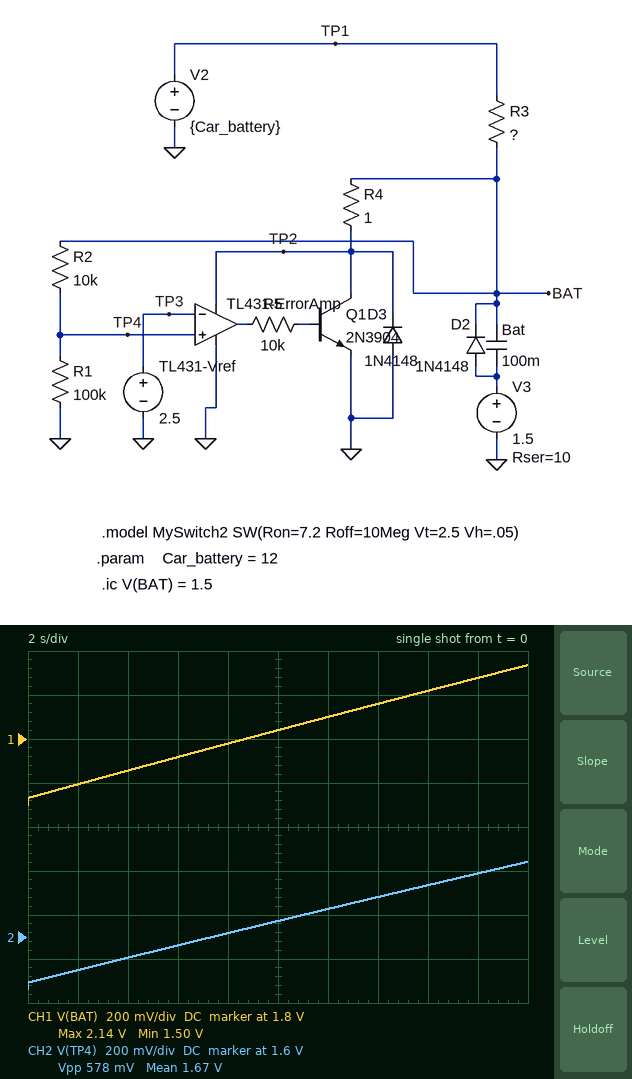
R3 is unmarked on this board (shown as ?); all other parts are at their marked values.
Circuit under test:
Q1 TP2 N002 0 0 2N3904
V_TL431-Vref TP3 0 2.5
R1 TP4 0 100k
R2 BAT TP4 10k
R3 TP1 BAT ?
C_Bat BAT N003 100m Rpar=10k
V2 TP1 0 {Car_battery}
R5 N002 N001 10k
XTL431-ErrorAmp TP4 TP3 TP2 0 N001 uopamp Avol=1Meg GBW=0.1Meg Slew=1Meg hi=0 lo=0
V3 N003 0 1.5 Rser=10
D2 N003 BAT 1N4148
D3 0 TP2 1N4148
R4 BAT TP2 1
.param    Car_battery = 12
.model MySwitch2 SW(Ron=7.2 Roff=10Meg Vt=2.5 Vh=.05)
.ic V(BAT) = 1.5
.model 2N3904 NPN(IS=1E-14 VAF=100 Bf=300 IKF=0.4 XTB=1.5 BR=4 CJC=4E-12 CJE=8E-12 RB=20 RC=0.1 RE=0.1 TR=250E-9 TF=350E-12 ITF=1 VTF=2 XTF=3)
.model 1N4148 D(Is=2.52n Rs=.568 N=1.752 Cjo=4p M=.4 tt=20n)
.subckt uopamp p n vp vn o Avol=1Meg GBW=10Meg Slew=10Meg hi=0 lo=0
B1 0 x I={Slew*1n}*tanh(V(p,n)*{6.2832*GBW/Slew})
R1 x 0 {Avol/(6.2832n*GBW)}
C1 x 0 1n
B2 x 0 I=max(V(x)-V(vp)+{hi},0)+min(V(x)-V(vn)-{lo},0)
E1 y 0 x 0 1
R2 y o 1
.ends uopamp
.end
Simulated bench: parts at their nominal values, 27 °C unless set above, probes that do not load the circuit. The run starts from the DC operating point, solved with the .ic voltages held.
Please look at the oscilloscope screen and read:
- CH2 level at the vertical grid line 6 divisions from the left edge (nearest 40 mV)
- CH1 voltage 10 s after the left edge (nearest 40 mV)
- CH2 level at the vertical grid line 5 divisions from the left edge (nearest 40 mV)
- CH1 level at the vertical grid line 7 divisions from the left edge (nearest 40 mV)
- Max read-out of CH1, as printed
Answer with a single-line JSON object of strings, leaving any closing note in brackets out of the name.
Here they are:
{"CH2 level at the vertical grid line 6 divisions from the left edge": "1.72 V", "CH1 voltage 10 s after the left edge": "1.84 V", "CH2 level at the vertical grid line 5 divisions from the left edge": "1.68 V", "CH1 level at the vertical grid line 7 divisions from the left edge": "1.96 V", "Max read-out of CH1, as printed": "2.14 V"}
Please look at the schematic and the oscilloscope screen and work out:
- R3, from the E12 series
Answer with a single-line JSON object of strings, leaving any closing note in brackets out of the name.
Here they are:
{"R3, from the E12 series": "3.3 kΩ"}
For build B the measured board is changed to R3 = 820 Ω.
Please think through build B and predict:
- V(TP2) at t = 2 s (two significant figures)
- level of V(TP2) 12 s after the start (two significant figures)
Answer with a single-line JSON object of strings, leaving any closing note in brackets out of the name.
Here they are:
{"V(TP2) at t = 2 s": "1.9 V", "level of V(TP2) 12 s after the start": "2.7 V"}
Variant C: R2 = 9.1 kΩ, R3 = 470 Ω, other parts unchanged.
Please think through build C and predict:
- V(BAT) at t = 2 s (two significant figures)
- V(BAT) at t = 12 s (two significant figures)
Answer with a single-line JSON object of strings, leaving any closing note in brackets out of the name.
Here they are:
{"V(BAT) at t = 2 s": "2.1 V", "V(BAT) at t = 12 s": "2.7 V"}
